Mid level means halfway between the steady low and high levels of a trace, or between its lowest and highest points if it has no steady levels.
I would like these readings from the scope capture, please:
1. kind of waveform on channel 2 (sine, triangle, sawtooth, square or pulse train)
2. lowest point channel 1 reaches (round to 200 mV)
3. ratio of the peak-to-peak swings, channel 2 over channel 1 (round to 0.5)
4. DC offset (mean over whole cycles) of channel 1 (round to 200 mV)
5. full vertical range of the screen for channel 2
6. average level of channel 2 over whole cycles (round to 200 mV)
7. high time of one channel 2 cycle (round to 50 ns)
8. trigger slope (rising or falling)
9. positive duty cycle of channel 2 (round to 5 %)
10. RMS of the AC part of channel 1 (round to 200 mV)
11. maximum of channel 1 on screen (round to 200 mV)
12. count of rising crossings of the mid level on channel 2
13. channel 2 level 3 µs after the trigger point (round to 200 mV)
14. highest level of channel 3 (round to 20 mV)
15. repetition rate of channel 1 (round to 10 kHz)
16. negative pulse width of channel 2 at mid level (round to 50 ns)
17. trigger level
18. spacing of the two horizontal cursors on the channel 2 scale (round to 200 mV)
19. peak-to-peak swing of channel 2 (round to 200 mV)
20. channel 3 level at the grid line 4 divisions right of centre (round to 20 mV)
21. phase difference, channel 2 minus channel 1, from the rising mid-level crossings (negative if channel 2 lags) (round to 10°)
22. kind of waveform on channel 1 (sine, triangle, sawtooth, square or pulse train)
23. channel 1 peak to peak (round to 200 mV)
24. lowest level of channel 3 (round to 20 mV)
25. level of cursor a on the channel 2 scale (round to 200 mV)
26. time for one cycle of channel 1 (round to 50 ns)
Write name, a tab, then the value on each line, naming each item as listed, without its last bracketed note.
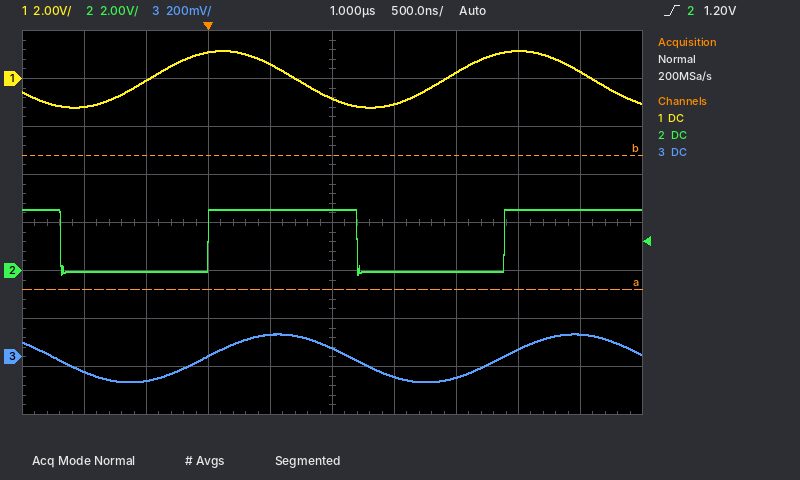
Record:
kind of waveform on channel 2	square
lowest point channel 1 reaches	-1.2 V
ratio of the peak-to-peak swings, channel 2 over channel 1	1.0
DC offset (mean over whole cycles) of channel 1	0.0 V
full vertical range of the screen for channel 2	16 V
average level of channel 2 over whole cycles	1.2 V
high time of one channel 2 cycle	1.20 µs
trigger slope	rising
positive duty cycle of channel 2	50 %
RMS of the AC part of channel 1	800 mV
maximum of channel 1 on screen	1.2 V
count of rising crossings of the mid level on channel 2	2
channel 2 level 3 µs after the trigger point	2.6 V
highest level of channel 3	100 mV
repetition rate of channel 1	420 kHz
negative pulse width of channel 2 at mid level	1.20 µs
trigger level	1.20 V
spacing of the two horizontal cursors on the channel 2 scale	5.6 V
peak-to-peak swing of channel 2	2.8 V
channel 3 level at the grid line 4 divisions right of centre	100 mV
phase difference, channel 2 minus channel 1, from the rising mid-level crossings (negative if channel 2 lags)	-70°
kind of waveform on channel 1	sine
channel 1 peak to peak	2.4 V
lowest level of channel 3	-100 mV
level of cursor a on the channel 2 scale	-800 mV
time for one cycle of channel 1	2.40 µs
